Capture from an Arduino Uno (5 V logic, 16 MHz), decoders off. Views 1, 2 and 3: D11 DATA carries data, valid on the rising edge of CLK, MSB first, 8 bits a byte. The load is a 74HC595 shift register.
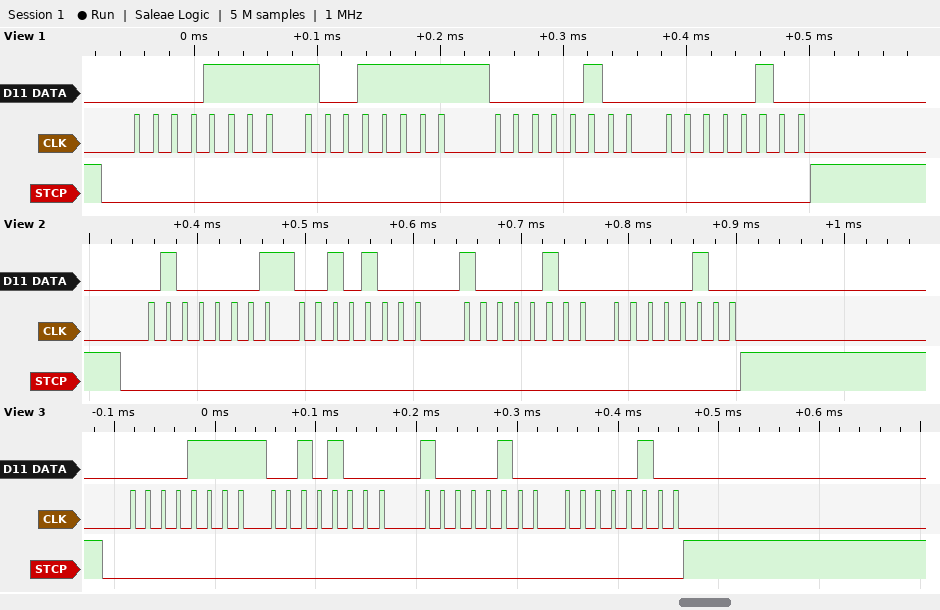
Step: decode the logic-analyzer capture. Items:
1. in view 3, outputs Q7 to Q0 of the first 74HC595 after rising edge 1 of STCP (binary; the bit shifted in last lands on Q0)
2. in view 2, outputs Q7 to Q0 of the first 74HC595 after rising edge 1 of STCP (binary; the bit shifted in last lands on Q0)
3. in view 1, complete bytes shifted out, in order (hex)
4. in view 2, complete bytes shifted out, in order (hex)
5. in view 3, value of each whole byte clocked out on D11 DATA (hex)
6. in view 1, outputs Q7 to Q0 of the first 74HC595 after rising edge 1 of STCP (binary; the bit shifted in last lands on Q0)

00000100
00000100
0F 9F 04 04
41 28 84 04
0F 28 84 04
00000100
